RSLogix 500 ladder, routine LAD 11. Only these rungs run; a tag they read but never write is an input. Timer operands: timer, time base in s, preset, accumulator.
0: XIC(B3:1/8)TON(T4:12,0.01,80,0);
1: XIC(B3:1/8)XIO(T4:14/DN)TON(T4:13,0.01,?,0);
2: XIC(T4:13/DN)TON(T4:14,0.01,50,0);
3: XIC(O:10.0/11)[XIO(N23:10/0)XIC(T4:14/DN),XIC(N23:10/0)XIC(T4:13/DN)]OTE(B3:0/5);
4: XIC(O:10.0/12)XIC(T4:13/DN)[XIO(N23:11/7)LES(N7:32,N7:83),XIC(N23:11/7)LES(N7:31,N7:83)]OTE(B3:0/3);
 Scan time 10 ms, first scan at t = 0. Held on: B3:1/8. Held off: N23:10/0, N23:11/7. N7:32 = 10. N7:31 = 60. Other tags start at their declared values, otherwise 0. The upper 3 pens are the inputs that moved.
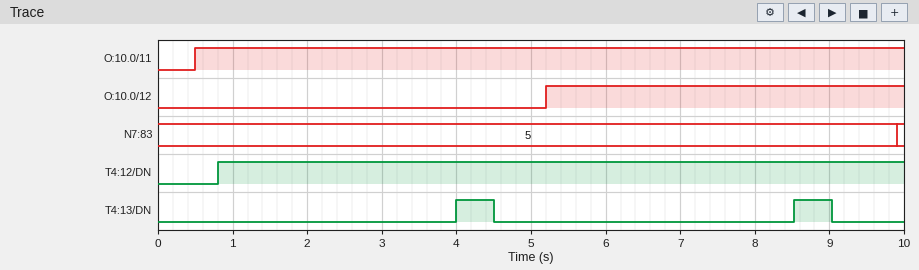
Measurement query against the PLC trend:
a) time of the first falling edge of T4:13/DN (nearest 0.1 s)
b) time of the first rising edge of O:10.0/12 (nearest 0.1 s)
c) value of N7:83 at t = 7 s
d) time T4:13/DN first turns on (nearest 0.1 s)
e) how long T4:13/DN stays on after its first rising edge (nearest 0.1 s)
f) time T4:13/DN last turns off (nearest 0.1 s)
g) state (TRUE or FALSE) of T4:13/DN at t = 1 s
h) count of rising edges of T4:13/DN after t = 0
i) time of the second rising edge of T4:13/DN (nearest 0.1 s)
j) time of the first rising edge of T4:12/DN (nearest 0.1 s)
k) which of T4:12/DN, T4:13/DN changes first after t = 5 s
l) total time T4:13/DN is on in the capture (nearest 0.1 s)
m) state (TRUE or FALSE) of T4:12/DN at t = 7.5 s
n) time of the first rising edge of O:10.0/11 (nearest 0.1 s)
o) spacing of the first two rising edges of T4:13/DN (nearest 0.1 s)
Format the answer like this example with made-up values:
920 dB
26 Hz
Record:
4.5 s
5.2 s
5
4.0 s
0.5 s
9.0 s
FALSE
2
8.5 s
0.8 s
T4:13/DN
1.0 s
TRUE
0.5 s
4.5 s
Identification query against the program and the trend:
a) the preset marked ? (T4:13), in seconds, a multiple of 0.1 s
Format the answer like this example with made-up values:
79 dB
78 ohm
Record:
4.0 s
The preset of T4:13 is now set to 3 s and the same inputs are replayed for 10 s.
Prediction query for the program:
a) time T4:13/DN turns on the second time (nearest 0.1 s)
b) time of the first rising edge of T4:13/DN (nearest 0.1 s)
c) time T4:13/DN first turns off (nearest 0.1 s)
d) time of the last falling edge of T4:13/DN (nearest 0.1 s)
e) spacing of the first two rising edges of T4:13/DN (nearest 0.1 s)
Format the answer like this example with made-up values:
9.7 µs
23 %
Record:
6.5 s
3.0 s
3.5 s
7.0 s
3.5 s
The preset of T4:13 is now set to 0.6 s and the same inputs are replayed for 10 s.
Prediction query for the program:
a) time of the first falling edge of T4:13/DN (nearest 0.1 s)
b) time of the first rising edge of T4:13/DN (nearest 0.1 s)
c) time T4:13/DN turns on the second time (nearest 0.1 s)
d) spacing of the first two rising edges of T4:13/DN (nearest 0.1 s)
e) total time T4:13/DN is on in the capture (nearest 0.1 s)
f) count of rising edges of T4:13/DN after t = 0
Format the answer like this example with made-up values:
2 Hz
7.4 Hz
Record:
1.1 s
0.6 s
1.7 s
1.1 s
4.5 s
9
